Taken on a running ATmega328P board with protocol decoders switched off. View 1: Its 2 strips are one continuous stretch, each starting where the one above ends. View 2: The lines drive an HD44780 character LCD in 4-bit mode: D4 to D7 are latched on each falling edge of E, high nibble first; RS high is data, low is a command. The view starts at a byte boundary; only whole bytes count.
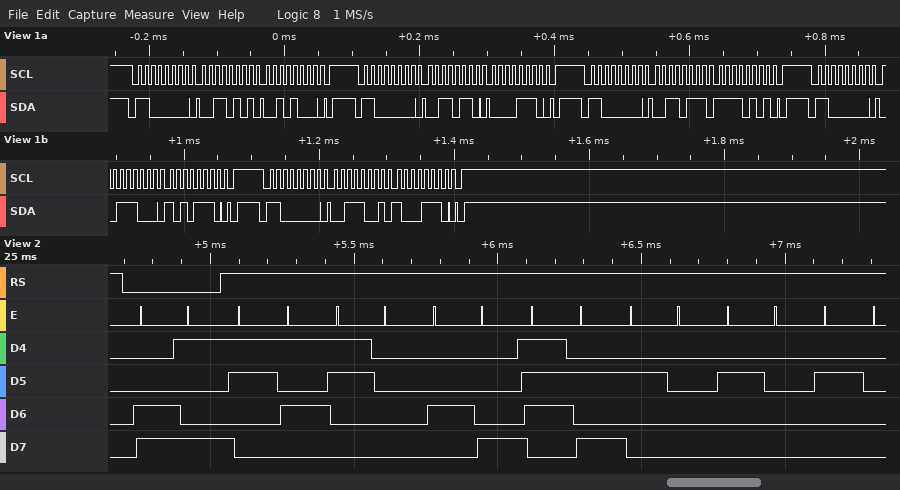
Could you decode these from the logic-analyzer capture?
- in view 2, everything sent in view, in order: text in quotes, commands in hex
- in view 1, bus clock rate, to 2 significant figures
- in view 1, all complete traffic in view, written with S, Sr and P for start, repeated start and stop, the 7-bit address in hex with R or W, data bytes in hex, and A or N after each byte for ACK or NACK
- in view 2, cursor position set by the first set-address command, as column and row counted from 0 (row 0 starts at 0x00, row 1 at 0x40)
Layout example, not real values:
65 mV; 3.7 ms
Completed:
0xC9 "50Hz   "; 100 kHz; S 60W A 35 A 28 A P S 60W A 36 A 0E A P S 60W A 37 A F5 A P S 60W A 38 A AE A P S 60W A 39 A 8E A P; column 9, row 1
